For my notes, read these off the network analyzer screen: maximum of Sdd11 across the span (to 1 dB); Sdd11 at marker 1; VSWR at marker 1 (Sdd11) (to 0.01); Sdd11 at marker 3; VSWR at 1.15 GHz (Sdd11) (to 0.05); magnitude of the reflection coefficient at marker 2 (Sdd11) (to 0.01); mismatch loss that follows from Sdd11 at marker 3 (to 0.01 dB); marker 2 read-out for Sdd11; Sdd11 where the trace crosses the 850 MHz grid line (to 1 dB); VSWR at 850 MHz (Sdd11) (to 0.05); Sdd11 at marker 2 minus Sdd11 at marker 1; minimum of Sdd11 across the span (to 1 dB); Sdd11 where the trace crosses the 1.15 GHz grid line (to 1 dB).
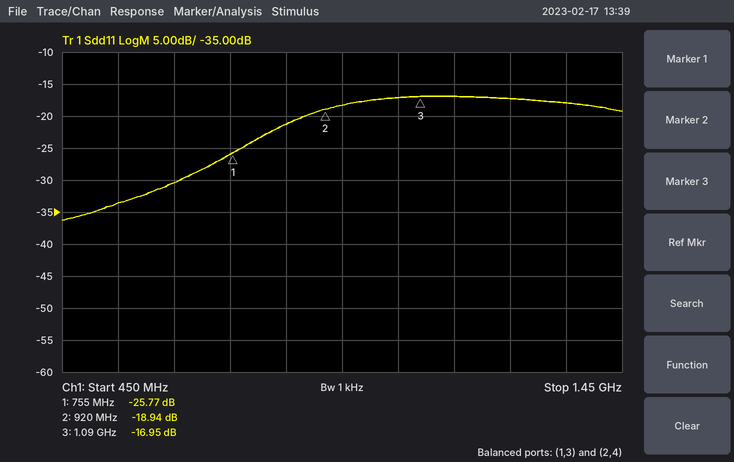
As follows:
-17 dB
-25.77 dB
1.11
-16.95 dB
1.35
0.11
0.09 dB
-18.94 dB
-21 dB
1.20
6.83 dB
-36 dB
-17 dB
